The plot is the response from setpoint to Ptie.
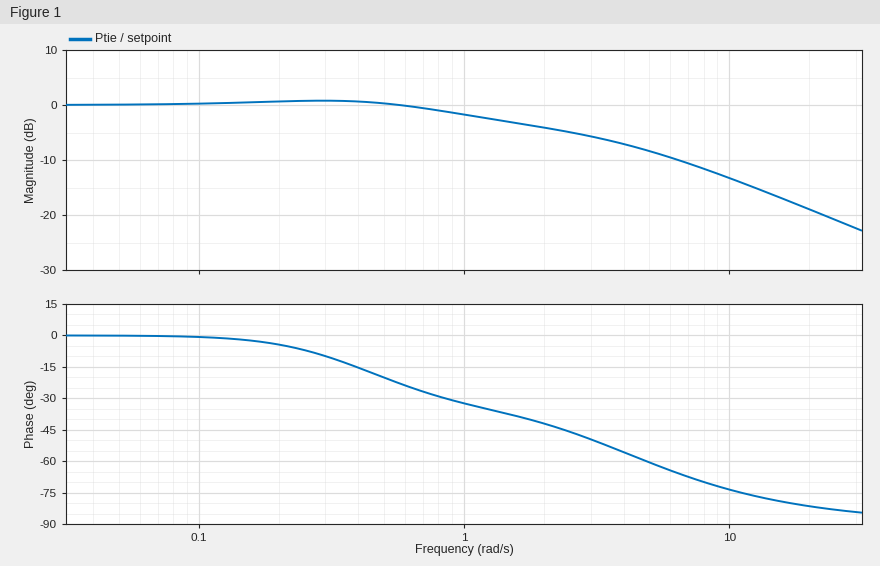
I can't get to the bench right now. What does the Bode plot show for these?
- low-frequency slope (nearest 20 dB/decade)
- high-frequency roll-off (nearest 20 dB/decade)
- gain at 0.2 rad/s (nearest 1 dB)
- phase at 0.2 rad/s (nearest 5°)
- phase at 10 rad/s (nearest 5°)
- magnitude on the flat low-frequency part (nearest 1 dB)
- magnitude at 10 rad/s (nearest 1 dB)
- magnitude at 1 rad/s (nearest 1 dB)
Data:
0 dB/decade
-20 dB/decade
1 dB
-5°
-75°
0 dB
-13 dB
-2 dB
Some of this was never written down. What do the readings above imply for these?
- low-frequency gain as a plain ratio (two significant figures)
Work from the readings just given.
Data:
1.0
